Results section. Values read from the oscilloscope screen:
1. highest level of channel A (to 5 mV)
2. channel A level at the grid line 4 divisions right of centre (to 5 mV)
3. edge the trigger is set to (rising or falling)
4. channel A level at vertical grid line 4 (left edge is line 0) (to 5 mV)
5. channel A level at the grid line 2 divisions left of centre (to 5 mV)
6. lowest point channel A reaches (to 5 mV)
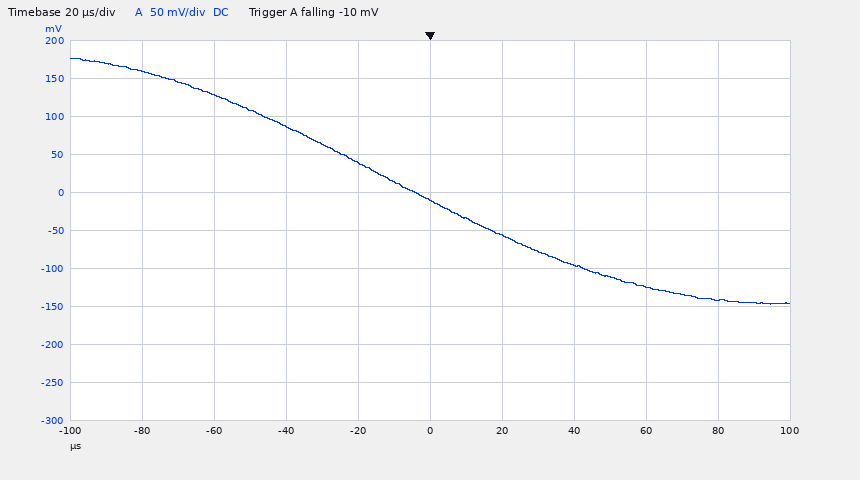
175 mV
-140 mV
falling
40 mV
85 mV
-145 mV
